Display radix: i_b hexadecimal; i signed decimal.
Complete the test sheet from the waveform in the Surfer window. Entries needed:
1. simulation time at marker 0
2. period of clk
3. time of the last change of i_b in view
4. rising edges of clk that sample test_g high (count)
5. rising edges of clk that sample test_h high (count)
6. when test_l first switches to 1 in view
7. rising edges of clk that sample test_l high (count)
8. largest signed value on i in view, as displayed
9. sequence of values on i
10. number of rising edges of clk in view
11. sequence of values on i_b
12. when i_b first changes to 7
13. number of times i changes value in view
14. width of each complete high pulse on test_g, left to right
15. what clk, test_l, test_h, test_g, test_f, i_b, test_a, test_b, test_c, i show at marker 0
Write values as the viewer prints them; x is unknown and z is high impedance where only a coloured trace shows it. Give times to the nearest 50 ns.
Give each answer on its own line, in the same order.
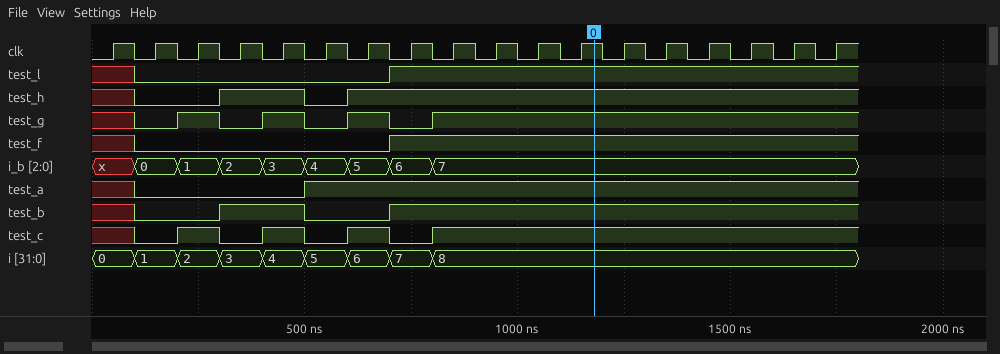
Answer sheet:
1200 ns
100 ns
800 ns
13
14
700 ns
11
8
0, 1, 2, 3, 4, 5, 6, 7, 8
18
x, 0, 1, 2, 3, 4, 5, 6, 7
800 ns
8
100 ns, 100 ns, 100 ns
clk=1, test_l=1, test_h=1, test_g=1, test_f=1, i_b=7, test_a=1, test_b=1, test_c=1, i=8
